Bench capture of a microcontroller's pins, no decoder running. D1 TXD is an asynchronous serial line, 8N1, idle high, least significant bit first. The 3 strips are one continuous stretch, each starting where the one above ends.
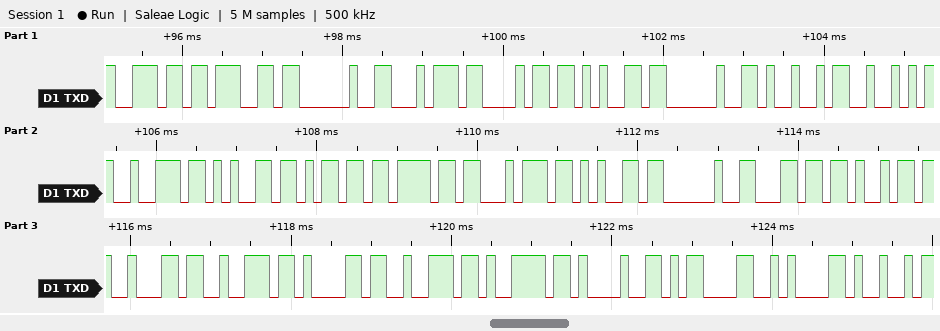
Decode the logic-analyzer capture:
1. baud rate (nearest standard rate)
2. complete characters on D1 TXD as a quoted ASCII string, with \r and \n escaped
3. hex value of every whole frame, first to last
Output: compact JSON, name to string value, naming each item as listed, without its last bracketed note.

{"baud rate": "9600 baud", "complete characters on D1 TXD as a quoted ASCII string, with \\r and \\n escaped": "\"ng the IRremote library!\\r\\nI\"", "hex value of every whole frame, first to last": "6E 67 20 74 68 65 20 49 52 72 65 6D 6F 74 65 20 6C 69 62 72 61 72 79 21 0D 0A 49"}
